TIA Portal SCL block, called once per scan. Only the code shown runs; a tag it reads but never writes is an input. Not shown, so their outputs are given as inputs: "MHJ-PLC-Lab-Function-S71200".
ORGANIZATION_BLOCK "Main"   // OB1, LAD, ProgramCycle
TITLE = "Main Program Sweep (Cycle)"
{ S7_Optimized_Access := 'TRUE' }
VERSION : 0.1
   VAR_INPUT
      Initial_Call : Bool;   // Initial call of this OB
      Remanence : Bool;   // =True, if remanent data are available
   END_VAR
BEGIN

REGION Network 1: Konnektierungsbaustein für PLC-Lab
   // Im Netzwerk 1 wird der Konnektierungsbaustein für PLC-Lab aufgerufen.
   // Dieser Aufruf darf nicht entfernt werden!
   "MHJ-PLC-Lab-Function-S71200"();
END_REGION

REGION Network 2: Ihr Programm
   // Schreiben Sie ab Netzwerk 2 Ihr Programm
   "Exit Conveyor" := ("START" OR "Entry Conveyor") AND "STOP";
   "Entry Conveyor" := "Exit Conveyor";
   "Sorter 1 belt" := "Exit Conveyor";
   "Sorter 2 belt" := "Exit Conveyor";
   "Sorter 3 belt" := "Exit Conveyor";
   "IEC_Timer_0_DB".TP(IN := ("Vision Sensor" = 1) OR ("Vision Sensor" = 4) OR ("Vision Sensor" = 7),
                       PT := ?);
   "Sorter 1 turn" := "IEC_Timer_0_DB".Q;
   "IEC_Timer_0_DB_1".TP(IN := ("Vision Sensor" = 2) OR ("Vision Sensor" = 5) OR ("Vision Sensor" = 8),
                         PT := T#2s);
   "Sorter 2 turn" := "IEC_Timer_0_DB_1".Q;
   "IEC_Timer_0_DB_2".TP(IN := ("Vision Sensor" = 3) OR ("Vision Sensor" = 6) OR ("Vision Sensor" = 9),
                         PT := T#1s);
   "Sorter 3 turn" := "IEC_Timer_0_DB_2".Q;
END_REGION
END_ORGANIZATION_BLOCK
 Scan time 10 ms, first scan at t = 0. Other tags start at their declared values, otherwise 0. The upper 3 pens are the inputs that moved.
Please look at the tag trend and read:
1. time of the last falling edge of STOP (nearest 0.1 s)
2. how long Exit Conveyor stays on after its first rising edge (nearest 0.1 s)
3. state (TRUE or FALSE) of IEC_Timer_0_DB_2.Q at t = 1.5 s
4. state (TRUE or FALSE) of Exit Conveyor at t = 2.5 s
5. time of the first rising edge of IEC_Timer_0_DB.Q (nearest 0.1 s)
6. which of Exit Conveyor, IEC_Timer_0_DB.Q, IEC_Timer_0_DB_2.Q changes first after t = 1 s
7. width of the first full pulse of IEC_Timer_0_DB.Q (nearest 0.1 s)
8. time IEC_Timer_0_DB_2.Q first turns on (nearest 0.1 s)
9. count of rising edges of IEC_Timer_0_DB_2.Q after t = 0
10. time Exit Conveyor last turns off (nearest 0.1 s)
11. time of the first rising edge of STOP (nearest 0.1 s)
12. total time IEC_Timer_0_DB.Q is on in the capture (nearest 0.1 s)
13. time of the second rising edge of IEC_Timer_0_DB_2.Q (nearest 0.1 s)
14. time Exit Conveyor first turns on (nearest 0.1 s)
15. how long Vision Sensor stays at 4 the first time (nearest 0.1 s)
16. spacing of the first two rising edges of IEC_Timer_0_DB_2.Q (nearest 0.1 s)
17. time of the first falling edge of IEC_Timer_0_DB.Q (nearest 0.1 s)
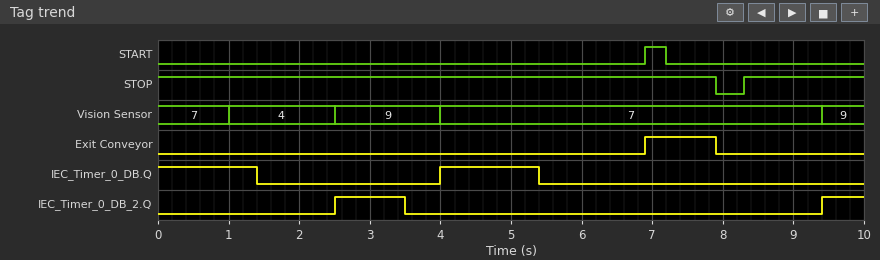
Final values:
7.9 s
1.0 s
FALSE
FALSE
4.0 s
IEC_Timer_0_DB.Q
1.4 s
2.5 s
2
7.9 s
8.3 s
2.8 s
9.4 s
6.9 s
1.5 s
6.9 s
1.4 s
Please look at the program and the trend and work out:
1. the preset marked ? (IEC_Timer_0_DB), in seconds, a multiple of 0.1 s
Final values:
1.4 s
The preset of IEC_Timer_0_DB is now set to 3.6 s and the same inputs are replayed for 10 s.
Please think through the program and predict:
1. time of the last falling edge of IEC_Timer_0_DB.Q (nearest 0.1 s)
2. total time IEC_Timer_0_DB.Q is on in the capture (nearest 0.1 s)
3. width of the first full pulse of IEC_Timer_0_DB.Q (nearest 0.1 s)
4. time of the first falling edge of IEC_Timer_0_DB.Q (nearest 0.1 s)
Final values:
7.6 s
7.2 s
3.6 s
3.6 s
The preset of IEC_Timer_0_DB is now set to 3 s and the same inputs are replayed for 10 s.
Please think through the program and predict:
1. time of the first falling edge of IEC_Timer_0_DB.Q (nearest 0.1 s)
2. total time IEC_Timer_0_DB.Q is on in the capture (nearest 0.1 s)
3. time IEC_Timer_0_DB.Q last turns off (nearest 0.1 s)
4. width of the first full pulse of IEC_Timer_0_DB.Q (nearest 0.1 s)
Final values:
3.0 s
6.0 s
7.0 s
3.0 s
